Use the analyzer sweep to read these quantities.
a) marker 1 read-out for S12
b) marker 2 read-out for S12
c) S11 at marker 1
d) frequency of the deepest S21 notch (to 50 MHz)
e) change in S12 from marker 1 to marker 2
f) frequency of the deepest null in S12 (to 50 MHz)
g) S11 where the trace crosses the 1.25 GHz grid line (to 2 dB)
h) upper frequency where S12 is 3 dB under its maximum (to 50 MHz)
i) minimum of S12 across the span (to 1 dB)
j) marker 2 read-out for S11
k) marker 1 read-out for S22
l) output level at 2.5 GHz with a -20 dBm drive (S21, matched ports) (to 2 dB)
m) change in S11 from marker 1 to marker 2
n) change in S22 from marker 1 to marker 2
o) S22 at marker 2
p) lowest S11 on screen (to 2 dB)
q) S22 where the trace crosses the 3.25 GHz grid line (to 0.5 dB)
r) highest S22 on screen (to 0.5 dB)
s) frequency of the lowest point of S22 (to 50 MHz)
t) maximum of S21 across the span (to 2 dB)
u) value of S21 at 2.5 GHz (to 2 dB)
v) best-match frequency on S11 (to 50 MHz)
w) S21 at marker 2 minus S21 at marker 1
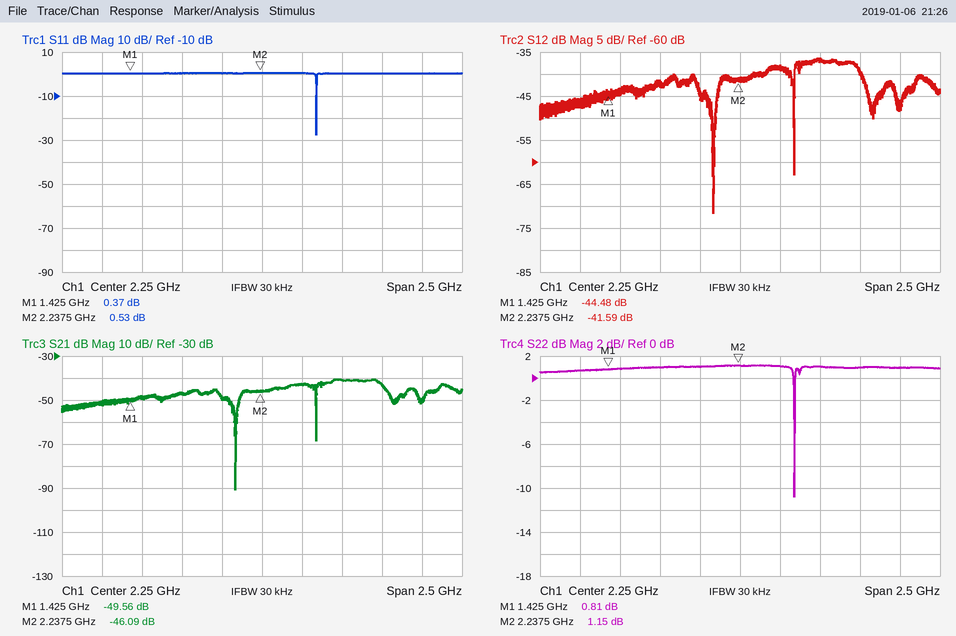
-44.48 dB
-41.59 dB
0.37 dB
2.10 GHz
2.89 dB
2.10 GHz
0 dB
3.00 GHz
-72 dB
0.53 dB
0.81 dB
-62 dBm
0.16 dB
0.34 dB
1.15 dB
-28 dB
1.0 dB
1.0 dB
2.60 GHz
-40 dB
-42 dB
2.60 GHz
3.47 dB
